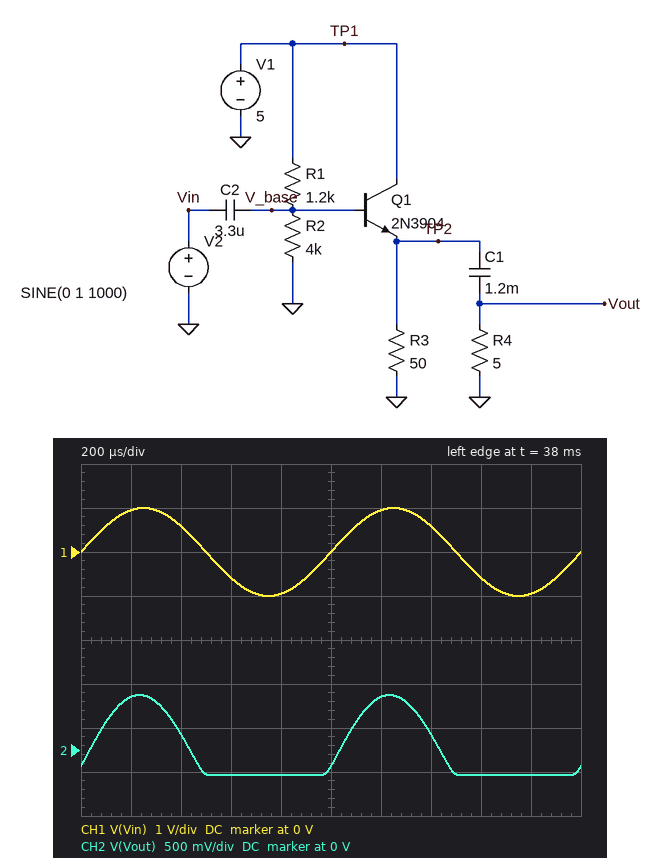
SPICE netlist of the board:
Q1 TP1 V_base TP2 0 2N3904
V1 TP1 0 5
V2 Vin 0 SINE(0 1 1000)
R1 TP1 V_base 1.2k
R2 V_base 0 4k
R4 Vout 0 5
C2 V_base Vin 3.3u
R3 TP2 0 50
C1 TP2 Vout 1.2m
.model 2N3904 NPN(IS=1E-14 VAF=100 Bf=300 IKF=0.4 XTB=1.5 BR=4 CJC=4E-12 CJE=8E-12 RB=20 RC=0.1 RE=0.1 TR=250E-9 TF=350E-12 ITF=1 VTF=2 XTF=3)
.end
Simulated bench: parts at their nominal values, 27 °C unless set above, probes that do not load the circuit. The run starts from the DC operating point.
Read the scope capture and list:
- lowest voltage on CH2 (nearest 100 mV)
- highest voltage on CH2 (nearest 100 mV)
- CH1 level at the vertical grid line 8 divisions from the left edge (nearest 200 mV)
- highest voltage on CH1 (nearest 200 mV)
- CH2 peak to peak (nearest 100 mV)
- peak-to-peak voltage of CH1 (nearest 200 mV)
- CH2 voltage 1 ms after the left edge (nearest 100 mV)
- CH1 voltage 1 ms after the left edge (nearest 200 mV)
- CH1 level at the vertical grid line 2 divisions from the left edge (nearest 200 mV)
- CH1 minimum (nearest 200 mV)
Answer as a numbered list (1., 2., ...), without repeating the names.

1. -300 mV
2. 600 mV
3. -600 mV
4. 1.0 V
5. 900 mV
6. 2.0 V
7. -200 mV
8. 0 V
9. 600 mV
10. -1.0 V
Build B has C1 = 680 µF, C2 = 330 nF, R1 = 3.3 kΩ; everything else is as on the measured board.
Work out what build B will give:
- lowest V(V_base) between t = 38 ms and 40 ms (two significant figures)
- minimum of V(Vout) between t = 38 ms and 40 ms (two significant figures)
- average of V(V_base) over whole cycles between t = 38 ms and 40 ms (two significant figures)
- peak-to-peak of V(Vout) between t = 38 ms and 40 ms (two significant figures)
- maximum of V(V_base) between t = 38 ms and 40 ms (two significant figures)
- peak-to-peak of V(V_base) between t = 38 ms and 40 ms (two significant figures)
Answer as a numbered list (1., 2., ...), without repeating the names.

1. 1.5 V
2. -190 mV
3. 2.4 V
4. 660 mV
5. 3.3 V
6. 1.8 V
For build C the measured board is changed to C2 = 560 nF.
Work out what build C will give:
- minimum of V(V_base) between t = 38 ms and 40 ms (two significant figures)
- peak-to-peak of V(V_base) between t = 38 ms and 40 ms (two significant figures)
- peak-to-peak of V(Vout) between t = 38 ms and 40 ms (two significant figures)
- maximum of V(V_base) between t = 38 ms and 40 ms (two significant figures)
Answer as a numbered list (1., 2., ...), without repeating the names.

1. 2.7 V
2. 1.8 V
3. 860 mV
4. 4.5 V
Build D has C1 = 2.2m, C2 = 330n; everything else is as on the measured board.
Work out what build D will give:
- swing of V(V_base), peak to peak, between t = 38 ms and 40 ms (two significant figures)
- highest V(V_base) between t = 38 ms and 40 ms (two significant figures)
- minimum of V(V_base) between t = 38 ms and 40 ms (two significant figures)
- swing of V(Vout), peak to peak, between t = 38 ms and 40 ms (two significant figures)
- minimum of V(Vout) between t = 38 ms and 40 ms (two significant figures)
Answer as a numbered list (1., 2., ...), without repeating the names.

1. 1.6 V
2. 4.4 V
3. 2.8 V
4. 810 mV
5. -270 mV
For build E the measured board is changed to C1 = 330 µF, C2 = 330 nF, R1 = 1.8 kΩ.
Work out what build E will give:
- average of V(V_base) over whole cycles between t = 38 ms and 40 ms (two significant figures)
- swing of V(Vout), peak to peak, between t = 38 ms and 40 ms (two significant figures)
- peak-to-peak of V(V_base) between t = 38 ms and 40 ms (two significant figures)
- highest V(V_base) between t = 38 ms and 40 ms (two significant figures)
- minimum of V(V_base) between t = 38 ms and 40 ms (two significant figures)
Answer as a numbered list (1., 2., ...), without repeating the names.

1. 3.2 V
2. 750 mV
3. 1.7 V
4. 4.0 V
5. 2.3 V
